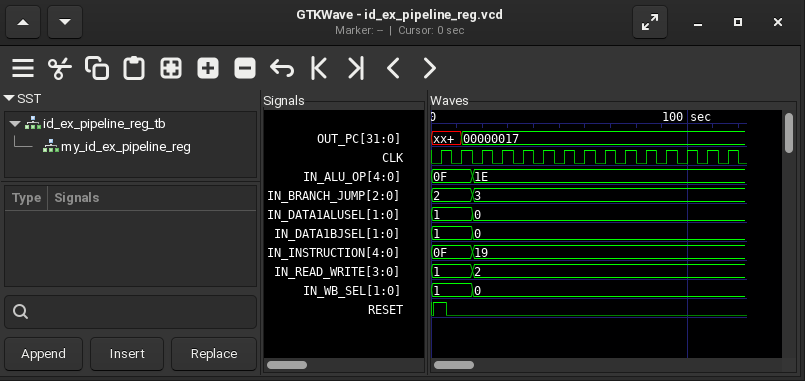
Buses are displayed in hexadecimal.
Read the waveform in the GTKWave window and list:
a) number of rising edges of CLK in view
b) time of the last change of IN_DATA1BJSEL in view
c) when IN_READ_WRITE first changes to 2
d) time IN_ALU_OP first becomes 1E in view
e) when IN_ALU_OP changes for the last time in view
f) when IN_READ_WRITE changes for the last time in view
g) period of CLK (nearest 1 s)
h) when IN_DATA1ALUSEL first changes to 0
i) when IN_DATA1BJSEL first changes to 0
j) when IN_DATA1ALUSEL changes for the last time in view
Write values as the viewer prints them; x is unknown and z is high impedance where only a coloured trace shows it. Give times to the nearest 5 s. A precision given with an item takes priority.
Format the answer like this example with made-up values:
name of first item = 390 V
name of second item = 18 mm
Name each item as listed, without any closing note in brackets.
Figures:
number of rising edges of CLK in view = 15
time of the last change of IN_DATA1BJSEL in view = 15 s
when IN_READ_WRITE first changes to 2 = 15 s
time IN_ALU_OP first becomes 1E in view = 15 s
when IN_ALU_OP changes for the last time in view = 15 s
when IN_READ_WRITE changes for the last time in view = 15 s
period of CLK = 8 s
when IN_DATA1ALUSEL first changes to 0 = 15 s
when IN_DATA1BJSEL first changes to 0 = 15 s
when IN_DATA1ALUSEL changes for the last time in view = 15 s
